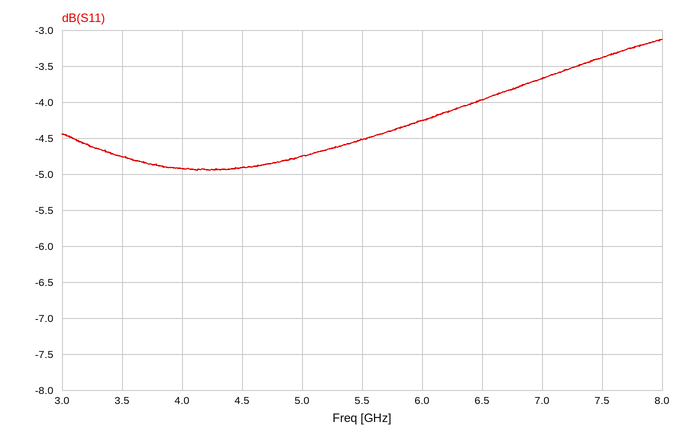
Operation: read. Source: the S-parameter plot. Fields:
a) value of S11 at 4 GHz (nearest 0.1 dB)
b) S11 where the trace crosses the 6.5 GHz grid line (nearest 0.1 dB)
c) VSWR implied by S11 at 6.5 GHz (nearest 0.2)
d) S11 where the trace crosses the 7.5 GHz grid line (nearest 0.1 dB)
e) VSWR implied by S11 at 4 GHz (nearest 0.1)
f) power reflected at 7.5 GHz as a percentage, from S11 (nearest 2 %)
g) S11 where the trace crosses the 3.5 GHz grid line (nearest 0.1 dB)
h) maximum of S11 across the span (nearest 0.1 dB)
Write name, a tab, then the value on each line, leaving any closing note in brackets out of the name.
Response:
value of S11 at 4 GHz	-4.9 dB
S11 where the trace crosses the 6.5 GHz grid line	-4.0 dB
VSWR implied by S11 at 6.5 GHz	4.4
S11 where the trace crosses the 7.5 GHz grid line	-3.4 dB
VSWR implied by S11 at 4 GHz	3.6
power reflected at 7.5 GHz as a percentage, from S11	46 %
S11 where the trace crosses the 3.5 GHz grid line	-4.8 dB
maximum of S11 across the span	-3.1 dB
